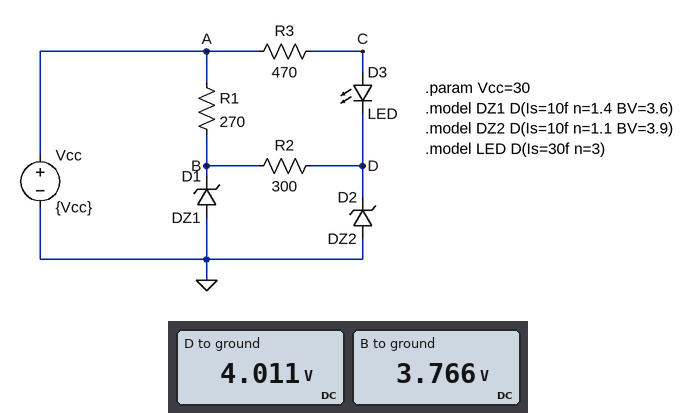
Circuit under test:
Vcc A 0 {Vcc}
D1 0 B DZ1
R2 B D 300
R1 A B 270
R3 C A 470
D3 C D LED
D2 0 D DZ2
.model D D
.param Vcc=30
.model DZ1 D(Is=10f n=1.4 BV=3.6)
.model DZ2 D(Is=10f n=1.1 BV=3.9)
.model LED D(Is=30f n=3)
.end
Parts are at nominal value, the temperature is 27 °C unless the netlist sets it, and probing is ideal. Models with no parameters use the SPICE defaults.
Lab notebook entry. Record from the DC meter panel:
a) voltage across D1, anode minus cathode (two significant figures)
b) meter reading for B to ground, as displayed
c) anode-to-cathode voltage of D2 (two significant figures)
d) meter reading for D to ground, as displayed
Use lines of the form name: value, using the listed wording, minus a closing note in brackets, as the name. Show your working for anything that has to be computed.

voltage across D1, anode minus cathode: 0 V - 3.766 V = -3.8 V
meter reading for B to ground, as displayed: 3.766 V
anode-to-cathode voltage of D2: 0 V - 4.011 V = -4.0 V
meter reading for D to ground, as displayed: 4.011 V
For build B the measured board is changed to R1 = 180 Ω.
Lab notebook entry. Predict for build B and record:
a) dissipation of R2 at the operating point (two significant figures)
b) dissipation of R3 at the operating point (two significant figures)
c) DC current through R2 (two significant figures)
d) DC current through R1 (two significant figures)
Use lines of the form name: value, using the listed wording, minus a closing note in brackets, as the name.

dissipation of R2 at the operating point: 180 µW
dissipation of R3 at the operating point: 1.2 W
DC current through R2: 770 µA
DC current through R1: 150 mA
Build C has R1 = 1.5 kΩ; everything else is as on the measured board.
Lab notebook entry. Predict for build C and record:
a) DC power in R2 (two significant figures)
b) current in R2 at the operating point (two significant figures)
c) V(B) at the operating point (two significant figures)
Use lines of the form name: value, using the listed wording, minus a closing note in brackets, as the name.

DC power in R2: 310 µW
current in R2 at the operating point: 1.0 mA
V(B) at the operating point: 3.7 V
